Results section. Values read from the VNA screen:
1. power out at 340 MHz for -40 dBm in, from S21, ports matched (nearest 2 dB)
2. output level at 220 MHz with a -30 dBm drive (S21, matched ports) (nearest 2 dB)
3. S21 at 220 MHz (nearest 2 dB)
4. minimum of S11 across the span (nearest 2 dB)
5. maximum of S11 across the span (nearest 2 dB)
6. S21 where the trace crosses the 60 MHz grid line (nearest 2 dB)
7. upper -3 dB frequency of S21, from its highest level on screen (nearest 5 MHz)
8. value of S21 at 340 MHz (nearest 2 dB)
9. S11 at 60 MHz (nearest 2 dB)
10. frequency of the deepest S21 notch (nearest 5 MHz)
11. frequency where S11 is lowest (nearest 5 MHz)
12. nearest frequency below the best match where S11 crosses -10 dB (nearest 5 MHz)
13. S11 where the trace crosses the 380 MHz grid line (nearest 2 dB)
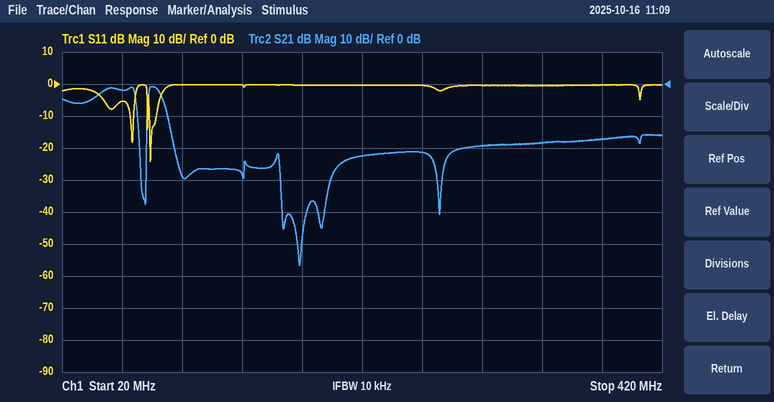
-58 dBm
-52 dBm
-22 dB
-24 dB
0 dB
-2 dB
85 MHz
-18 dB
-6 dB
180 MHz
80 MHz
80 MHz
0 dB
